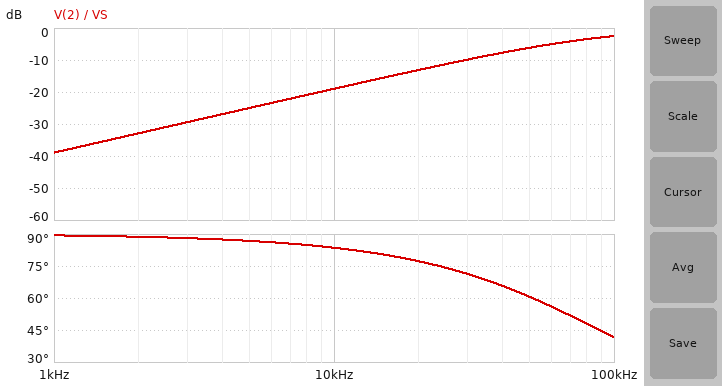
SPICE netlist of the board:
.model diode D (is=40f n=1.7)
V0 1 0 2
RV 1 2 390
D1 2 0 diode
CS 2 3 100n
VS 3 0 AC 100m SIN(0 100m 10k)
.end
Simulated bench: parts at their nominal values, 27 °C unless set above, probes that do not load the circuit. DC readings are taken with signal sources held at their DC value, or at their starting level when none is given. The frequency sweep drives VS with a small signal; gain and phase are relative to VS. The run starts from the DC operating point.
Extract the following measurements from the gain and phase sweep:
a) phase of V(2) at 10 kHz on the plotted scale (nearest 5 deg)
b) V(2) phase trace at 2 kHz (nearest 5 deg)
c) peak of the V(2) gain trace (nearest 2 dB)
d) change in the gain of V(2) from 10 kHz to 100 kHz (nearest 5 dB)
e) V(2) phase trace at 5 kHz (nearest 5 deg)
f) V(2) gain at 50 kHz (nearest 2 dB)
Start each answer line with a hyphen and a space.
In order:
- 85 deg
- 90 deg
- -2 dB
- 15 dB
- 85 deg
- -6 dB
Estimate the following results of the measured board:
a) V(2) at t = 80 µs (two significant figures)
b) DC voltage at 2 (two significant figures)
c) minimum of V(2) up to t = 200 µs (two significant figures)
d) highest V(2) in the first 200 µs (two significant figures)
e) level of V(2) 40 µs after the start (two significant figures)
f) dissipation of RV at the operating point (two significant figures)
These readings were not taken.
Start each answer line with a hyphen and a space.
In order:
- 1.1 V
- 1.1 V
- 1.1 V
- 1.1 V
- 1.1 V
- 2.1 mW
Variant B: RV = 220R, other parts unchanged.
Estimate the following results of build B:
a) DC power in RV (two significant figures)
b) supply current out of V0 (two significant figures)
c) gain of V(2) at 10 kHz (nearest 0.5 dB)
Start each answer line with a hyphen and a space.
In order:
- 3.6 mW
- 4.0 mA
- -23.5 dB
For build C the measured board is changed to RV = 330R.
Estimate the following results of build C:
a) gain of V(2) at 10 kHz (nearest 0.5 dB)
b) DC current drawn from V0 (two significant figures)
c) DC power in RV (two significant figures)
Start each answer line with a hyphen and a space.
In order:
- -20.5 dB
- 2.7 mA
- 2.5 mW
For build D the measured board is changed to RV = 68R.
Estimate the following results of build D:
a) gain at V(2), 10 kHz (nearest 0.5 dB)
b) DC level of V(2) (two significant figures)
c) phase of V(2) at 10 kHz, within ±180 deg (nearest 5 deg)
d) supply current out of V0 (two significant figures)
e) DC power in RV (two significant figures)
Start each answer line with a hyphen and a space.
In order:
- -33.5 dB
- 1.2 V
- 90 deg
- 12 mA
- 10 mW
